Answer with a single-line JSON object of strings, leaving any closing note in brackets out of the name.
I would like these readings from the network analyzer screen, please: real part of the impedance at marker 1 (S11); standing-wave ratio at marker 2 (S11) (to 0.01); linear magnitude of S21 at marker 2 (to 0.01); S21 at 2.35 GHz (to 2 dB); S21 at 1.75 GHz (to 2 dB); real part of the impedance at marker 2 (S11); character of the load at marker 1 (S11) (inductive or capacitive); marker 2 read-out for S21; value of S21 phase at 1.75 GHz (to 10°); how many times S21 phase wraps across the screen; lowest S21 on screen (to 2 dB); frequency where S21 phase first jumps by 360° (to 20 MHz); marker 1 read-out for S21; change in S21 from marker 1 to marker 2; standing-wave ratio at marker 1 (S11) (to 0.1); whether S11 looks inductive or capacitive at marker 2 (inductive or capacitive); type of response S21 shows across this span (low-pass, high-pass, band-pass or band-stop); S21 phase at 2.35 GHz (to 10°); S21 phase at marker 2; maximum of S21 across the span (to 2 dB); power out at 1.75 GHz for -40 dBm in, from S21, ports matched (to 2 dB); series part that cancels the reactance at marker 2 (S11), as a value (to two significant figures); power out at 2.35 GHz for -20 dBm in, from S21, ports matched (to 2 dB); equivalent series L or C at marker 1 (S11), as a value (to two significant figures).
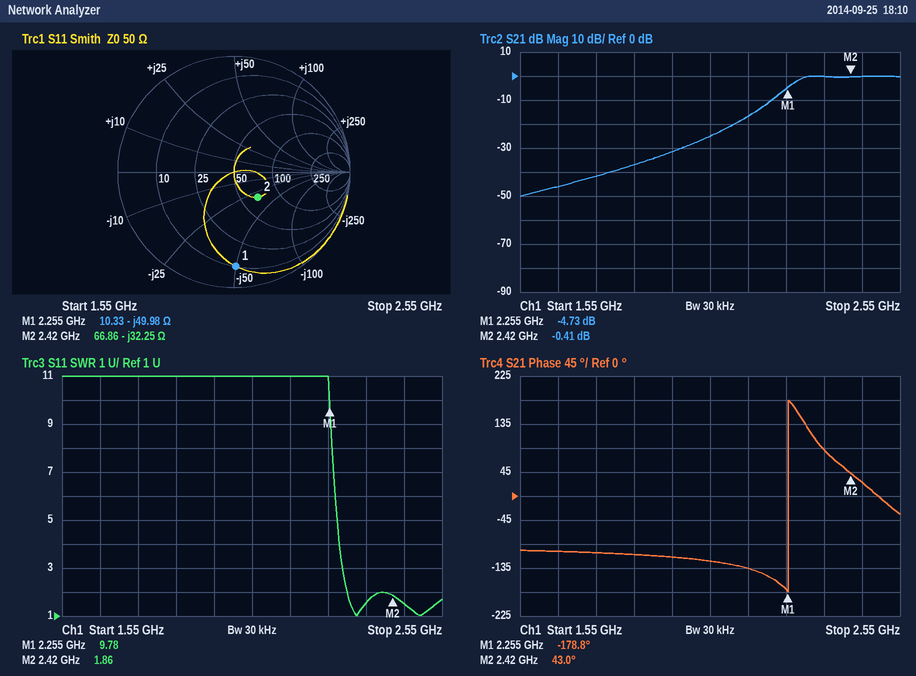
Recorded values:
{"real part of the impedance at marker 1": "10.33 Ω", "standing-wave ratio at marker 2 (S11)": "1.86", "linear magnitude of S21 at marker 2": "0.95", "S21 at 2.35 GHz": "0 dB", "S21 at 1.75 GHz": "-42 dB", "real part of the impedance at marker 2": "66.86 Ω", "character of the load at marker 1 (S11)": "capacitive", "marker 2 read-out for S21": "-0.41 dB", "value of S21 phase at 1.75 GHz": "-110°", "how many times S21 phase wraps across the screen": "1", "lowest S21 on screen": "-50 dB", "frequency where S21 phase first jumps by 360°": "2.26 GHz", "marker 1 read-out for S21": "-4.73 dB", "change in S21 from marker 1 to marker 2": "4.32 dB", "standing-wave ratio at marker 1 (S11)": "9.8", "whether S11 looks inductive or capacitive at marker 2": "capacitive", "type of response S21 shows across this span": "high-pass", "S21 phase at 2.35 GHz": "90°", "S21 phase at marker 2": "43.0°", "maximum of S21 across the span": "0 dB", "power out at 1.75 GHz for -40 dBm in, from S21, ports matched": "-82 dBm", "series part that cancels the reactance at marker 2 (S11), as a value": "2.1 nH", "power out at 2.35 GHz for -20 dBm in, from S21, ports matched": "-20 dBm", "equivalent series L or C at marker 1 (S11), as a value": "1.4 pF"}
